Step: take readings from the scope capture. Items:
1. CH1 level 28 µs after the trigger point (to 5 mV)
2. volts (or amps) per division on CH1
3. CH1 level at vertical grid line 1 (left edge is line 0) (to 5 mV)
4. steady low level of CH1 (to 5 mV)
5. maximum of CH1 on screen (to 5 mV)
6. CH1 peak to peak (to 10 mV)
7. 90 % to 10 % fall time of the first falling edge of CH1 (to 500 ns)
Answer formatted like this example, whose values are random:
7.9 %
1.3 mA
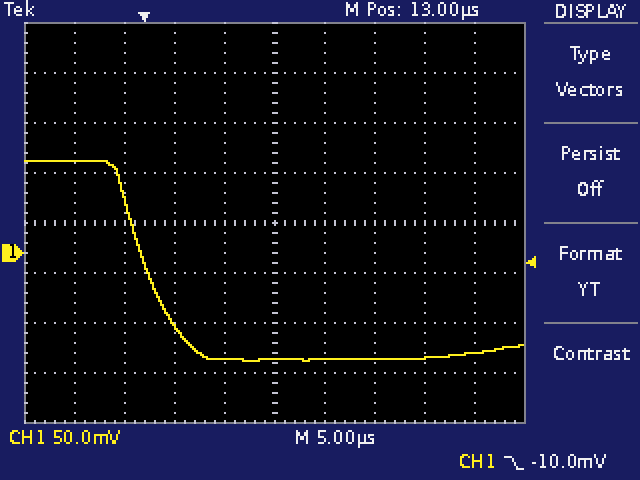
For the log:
-105 mV
50 mV
90 mV
-105 mV
90 mV
200 mV
6.5 µs
